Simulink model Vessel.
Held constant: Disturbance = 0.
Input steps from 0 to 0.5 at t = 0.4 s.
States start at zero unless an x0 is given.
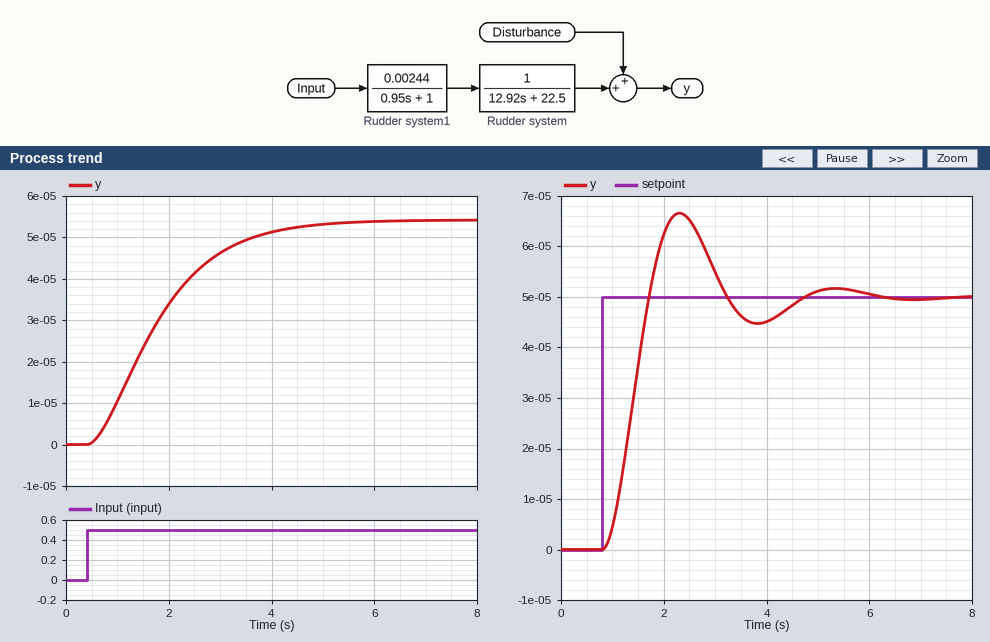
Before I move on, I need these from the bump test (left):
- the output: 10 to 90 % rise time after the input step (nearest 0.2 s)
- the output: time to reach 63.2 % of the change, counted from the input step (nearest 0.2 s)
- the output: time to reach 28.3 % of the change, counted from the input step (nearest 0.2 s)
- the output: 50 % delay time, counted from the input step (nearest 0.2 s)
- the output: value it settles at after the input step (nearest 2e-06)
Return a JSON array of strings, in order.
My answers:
["2.6 s", "1.6 s", "0.8 s", "1.2 s", "0.000054"]
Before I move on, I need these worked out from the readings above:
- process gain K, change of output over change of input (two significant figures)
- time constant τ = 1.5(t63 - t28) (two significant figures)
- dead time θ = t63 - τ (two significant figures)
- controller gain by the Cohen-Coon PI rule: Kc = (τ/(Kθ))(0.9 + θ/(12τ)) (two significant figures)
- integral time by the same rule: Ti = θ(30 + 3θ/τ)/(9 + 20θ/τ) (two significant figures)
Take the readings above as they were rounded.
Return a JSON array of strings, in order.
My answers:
["0.00011", "1.2 s", "0.40 s", "25000", "0.79 s"]
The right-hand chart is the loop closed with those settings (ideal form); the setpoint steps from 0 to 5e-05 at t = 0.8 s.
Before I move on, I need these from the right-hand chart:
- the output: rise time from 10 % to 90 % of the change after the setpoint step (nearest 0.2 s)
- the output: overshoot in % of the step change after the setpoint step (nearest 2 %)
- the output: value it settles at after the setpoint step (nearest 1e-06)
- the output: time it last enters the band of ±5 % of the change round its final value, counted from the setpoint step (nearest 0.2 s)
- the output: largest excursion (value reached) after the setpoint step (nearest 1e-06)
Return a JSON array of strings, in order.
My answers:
["0.6 s", "34 %", "0.000050", "3.6 s", "0.000067"]
